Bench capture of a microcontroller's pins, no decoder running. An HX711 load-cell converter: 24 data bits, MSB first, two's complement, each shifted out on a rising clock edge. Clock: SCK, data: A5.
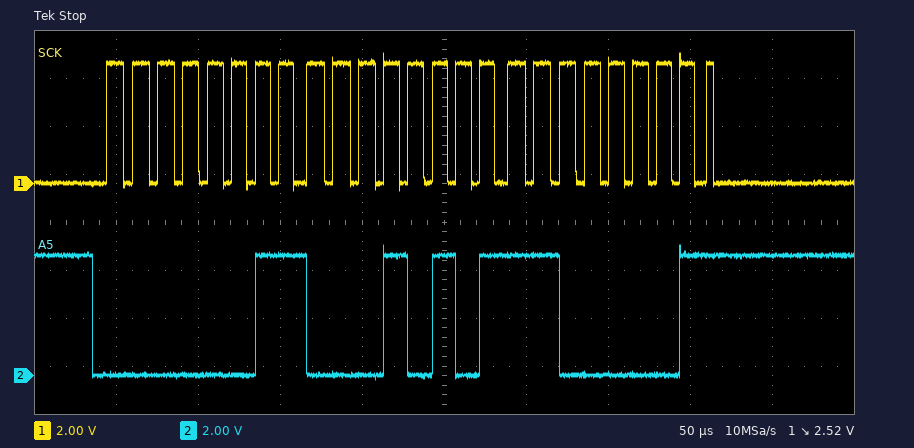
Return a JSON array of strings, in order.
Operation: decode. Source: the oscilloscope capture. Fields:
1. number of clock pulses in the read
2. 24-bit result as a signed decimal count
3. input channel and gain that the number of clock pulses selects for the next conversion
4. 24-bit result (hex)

["25", "202177", "channel A, gain 128", "0x0315C1"]
